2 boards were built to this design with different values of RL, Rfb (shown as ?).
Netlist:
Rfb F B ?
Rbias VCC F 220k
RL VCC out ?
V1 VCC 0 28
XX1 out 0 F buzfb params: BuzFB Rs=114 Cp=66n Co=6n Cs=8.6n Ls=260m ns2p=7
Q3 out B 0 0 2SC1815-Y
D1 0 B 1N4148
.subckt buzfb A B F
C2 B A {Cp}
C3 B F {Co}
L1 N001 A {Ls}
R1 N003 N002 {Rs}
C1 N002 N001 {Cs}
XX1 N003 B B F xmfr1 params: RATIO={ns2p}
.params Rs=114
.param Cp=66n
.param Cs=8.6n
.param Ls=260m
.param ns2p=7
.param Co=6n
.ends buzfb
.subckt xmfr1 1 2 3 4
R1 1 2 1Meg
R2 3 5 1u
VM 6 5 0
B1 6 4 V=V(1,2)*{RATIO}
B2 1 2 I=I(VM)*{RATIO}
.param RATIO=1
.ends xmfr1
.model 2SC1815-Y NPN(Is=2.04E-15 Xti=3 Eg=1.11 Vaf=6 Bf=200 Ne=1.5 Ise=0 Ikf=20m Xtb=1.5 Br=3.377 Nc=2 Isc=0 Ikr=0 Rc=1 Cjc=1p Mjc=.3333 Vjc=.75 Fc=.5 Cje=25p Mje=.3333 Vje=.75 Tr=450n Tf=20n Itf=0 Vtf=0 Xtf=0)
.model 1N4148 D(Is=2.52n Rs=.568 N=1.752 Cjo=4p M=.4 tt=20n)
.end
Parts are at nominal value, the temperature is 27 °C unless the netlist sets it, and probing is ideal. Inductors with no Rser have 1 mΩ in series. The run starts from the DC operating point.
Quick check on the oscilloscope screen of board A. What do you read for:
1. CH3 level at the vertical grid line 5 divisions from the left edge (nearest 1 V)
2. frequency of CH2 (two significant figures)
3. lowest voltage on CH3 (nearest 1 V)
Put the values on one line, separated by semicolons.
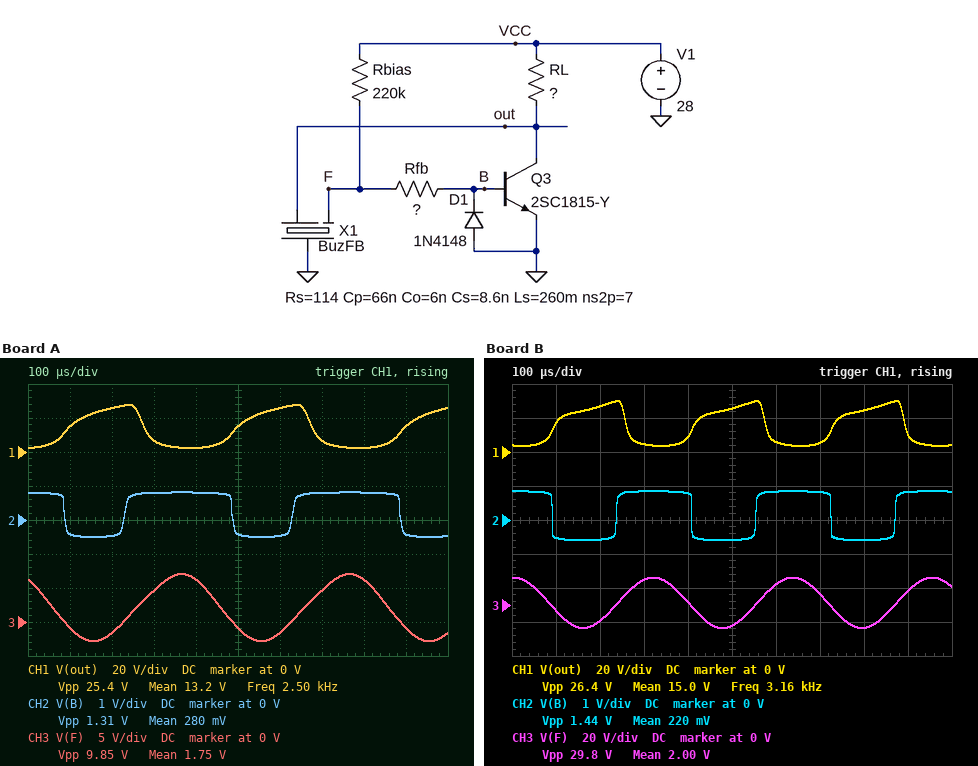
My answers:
-1 V; 2.5 kHz; -3 V
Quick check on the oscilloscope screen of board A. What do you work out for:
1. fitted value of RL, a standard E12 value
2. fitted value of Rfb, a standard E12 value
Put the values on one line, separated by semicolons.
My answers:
680 Ω; 15 kΩ
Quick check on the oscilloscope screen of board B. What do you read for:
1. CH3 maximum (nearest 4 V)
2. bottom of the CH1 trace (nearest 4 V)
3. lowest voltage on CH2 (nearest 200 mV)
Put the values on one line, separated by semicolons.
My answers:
16 V; 4 V; -600 mV
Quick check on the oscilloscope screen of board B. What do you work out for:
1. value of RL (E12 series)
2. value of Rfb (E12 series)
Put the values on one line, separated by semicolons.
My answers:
270 Ω; 10 kΩ
